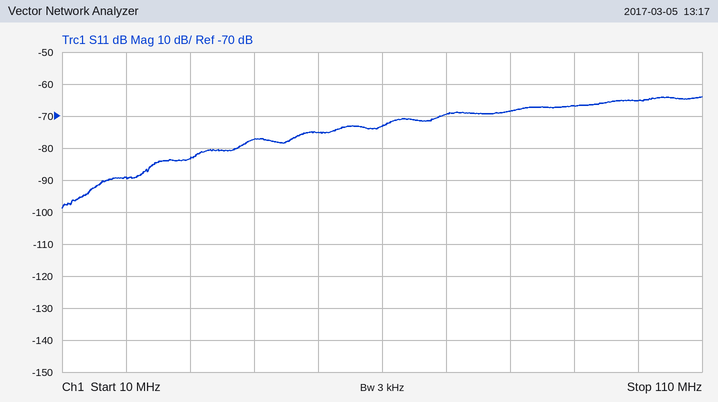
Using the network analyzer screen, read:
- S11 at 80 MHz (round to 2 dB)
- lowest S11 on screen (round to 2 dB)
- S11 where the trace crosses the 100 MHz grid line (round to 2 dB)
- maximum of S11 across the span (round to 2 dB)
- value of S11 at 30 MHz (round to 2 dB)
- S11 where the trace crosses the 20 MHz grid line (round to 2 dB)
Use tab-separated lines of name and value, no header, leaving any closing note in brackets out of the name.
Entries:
S11 at 80 MHz	-68 dB
lowest S11 on screen	-98 dB
S11 where the trace crosses the 100 MHz grid line	-66 dB
maximum of S11 across the span	-64 dB
value of S11 at 30 MHz	-84 dB
S11 where the trace crosses the 20 MHz grid line	-90 dB
